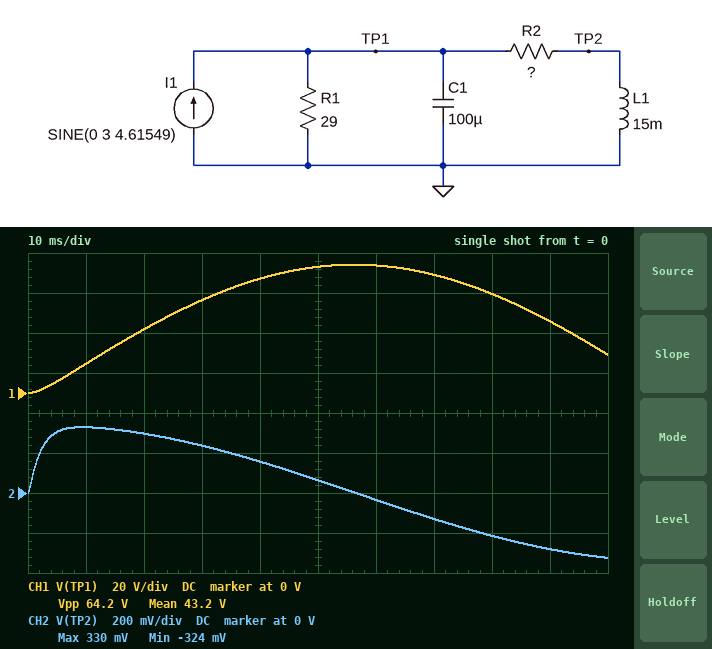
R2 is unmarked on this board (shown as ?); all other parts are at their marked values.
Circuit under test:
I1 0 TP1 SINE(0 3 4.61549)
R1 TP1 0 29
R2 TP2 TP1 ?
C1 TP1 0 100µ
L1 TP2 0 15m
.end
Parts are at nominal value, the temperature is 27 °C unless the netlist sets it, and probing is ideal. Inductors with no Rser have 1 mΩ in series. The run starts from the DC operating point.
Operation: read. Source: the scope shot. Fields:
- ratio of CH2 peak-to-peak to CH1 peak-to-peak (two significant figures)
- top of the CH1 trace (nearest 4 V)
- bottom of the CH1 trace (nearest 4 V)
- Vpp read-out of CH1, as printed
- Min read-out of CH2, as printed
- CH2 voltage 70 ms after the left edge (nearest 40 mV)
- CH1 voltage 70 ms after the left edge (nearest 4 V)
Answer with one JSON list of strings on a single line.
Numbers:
["0.010", "64 V", "0 V", "64.2 V", "-324 mV", "-120 mV", "60 V"]
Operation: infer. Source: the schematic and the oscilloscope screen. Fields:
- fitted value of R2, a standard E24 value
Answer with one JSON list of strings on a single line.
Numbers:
["82 Ω"]
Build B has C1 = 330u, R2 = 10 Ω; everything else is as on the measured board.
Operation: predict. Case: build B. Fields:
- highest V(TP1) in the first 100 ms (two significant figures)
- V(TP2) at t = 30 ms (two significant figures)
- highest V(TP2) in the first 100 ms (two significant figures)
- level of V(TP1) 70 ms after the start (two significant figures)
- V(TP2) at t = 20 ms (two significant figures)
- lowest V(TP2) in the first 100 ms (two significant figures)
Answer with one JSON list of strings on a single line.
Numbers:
["22 V", "690 mV", "990 mV", "20 V", "850 mV", "-920 mV"]
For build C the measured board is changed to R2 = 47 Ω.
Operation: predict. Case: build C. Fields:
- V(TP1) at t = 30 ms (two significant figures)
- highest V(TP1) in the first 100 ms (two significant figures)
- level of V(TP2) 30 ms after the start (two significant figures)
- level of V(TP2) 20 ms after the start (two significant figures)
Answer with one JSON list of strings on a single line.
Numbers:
["39 V", "54 V", "340 mV", "430 mV"]
